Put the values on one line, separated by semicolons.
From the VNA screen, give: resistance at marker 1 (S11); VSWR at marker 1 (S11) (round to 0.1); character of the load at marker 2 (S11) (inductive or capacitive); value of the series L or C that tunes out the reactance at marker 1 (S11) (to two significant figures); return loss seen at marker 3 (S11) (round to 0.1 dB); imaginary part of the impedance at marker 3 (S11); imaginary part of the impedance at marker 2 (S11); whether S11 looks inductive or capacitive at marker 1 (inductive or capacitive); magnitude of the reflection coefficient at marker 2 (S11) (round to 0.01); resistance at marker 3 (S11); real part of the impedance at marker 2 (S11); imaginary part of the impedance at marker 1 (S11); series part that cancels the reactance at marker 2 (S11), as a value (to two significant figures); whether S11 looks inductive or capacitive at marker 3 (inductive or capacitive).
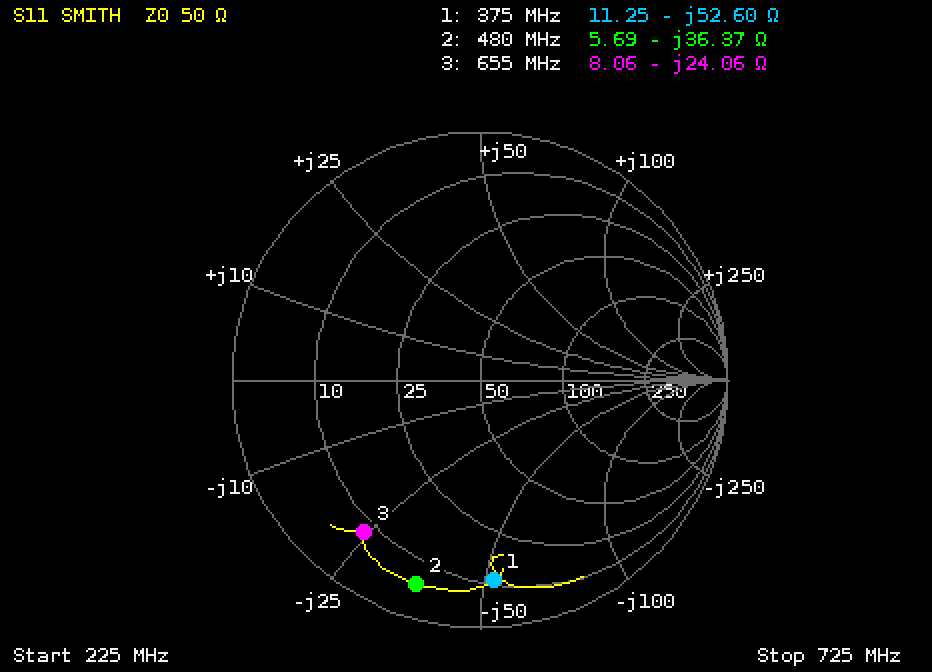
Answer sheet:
11.25 Ω; 9.5; capacitive; 22 nH; 2.3 dB; -24.06 Ω; -36.37 Ω; capacitive; 0.86; 8.06 Ω; 5.69 Ω; -52.60 Ω; 12 nH; capacitive
